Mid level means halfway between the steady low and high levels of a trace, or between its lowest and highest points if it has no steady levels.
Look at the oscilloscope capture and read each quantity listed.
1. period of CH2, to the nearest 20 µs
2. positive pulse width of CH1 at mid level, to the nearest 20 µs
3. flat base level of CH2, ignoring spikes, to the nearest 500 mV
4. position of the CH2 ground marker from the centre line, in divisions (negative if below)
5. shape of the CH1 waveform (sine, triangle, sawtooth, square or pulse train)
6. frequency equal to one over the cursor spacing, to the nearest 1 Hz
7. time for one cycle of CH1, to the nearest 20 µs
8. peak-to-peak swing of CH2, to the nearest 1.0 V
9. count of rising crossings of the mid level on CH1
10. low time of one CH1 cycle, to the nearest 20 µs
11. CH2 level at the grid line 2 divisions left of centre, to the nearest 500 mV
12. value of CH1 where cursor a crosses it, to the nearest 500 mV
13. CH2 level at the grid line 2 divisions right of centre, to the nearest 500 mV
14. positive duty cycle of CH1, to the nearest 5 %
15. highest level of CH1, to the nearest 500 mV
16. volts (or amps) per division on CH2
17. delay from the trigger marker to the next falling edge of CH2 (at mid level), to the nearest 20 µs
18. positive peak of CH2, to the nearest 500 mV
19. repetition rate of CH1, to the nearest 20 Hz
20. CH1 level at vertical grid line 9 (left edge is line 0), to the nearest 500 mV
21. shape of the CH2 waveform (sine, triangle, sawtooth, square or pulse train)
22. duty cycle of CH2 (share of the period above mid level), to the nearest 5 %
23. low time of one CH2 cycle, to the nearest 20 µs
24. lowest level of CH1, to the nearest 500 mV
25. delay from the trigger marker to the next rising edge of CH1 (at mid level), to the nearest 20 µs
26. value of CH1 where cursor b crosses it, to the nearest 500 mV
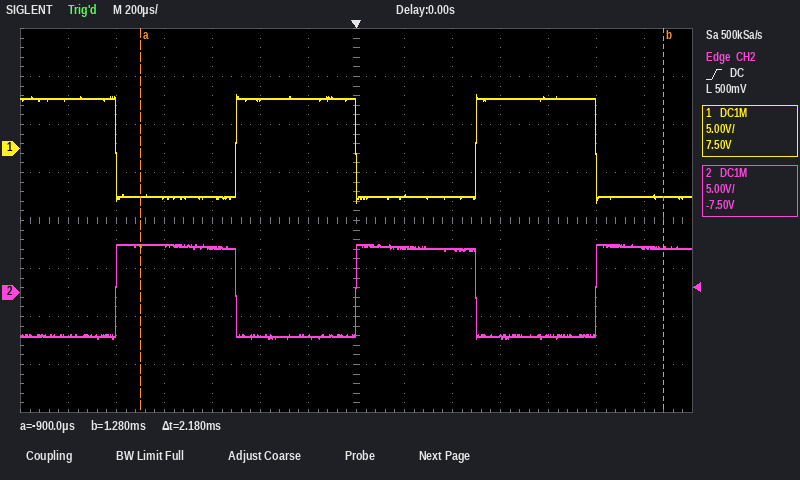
1.00 ms
500 µs
-4.5 V
-1.5 div
square
459 Hz
1.00 ms
10.0 V
2
500 µs
-4.5 V
-5.0 V
4.5 V
50 %
5.5 V
5 V
500 µs
5.0 V
1.00 kHz
-5.0 V
square
50 %
500 µs
-5.5 V
500 µs
-5.0 V
